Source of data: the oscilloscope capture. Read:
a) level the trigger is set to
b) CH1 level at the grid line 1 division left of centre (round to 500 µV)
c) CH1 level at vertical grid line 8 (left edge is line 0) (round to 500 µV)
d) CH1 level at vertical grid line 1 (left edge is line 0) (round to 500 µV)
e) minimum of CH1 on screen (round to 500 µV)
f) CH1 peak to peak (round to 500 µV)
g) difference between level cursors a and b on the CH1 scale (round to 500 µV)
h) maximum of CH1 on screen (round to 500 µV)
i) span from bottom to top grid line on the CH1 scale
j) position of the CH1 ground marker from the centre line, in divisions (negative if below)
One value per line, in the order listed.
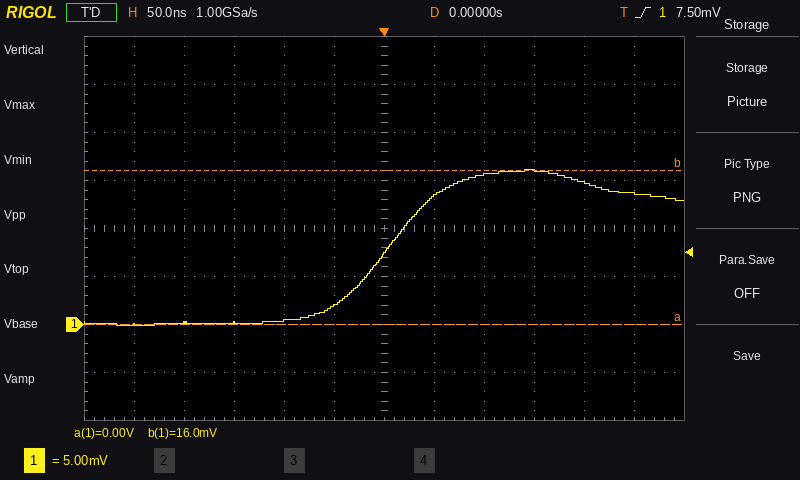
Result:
7.50 mV
2.0 mV
15.5 mV
0.0 mV
0.0 mV
16.0 mV
16.0 mV
16.0 mV
40 mV
-2.0 div
